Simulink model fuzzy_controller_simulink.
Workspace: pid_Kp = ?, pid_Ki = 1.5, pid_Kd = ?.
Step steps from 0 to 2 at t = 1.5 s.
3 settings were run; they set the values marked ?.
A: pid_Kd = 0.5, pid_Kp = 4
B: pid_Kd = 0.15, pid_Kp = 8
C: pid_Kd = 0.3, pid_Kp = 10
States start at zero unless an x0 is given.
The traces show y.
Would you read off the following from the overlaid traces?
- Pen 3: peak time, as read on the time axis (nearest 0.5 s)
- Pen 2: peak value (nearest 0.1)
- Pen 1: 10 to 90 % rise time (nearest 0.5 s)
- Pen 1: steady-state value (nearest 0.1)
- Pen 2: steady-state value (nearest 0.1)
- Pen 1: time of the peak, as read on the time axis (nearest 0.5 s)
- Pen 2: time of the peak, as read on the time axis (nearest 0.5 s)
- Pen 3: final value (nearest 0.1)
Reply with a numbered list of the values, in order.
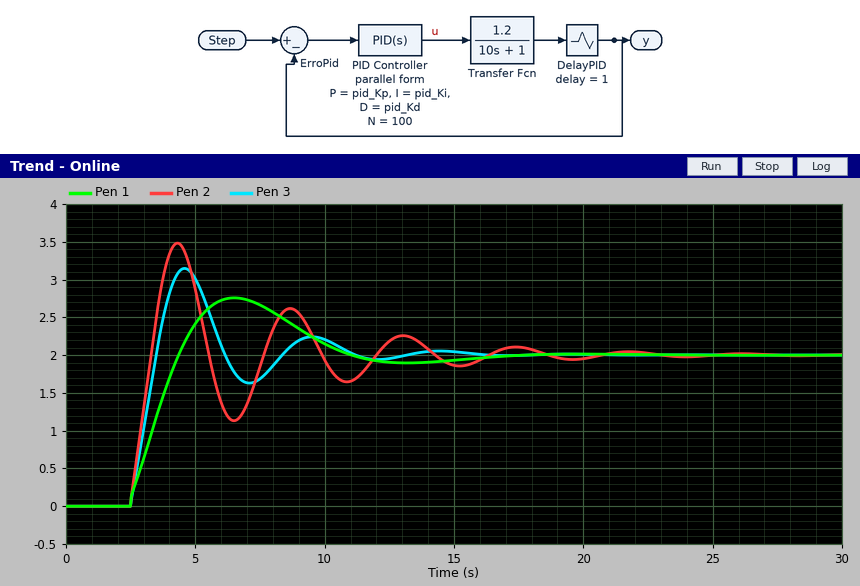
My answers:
1. 4.5 s
2. 3.5
3. 1.5 s
4. 2.0
5. 2.0
6. 6.5 s
7. 4.5 s
8. 2.0
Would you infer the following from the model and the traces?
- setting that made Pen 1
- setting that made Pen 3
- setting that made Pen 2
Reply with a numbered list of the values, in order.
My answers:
1. A
2. B
3. C
